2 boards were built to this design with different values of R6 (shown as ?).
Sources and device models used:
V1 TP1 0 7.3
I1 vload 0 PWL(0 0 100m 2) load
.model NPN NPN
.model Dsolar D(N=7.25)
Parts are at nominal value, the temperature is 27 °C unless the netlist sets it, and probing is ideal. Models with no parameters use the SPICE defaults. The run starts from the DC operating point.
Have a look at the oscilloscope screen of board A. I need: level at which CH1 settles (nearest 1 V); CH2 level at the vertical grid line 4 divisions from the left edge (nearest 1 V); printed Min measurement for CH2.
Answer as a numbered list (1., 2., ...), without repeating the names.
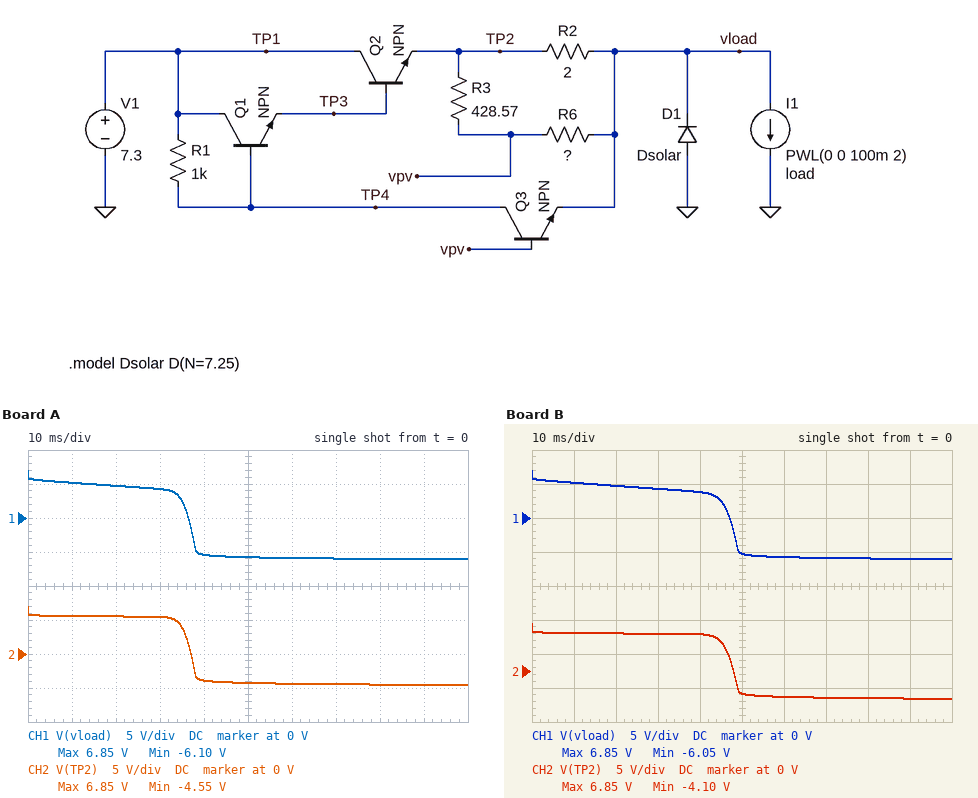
1. -6 V
2. -4 V
3. -4.55 V
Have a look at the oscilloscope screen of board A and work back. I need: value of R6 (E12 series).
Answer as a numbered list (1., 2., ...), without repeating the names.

1. 560 Ω
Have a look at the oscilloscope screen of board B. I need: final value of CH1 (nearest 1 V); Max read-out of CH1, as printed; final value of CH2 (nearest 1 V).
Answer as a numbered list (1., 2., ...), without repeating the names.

1. -6 V
2. 6.85 V
3. -4 V
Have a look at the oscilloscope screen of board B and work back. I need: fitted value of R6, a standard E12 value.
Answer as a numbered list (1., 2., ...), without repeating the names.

1. 330 Ω
